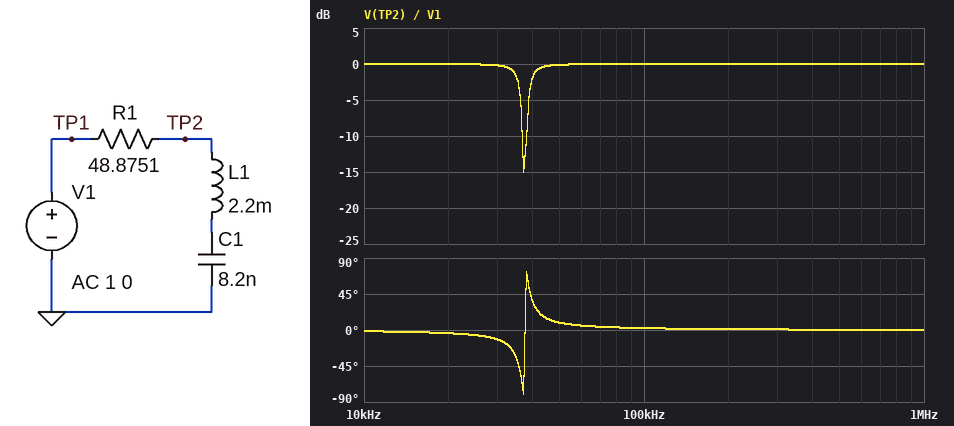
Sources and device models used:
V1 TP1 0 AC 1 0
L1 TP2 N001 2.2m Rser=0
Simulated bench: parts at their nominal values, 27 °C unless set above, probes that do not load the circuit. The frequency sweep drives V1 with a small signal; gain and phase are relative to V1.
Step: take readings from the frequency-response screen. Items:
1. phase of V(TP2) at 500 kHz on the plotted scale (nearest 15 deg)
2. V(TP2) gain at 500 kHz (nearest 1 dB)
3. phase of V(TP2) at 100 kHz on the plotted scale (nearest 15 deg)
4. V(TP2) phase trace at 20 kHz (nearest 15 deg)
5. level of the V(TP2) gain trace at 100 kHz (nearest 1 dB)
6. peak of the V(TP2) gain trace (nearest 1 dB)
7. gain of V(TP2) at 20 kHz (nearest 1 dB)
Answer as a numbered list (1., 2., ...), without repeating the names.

1. 0 deg
2. 0 dB
3. 0 deg
4. 0 deg
5. 0 dB
6. 0 dB
7. 0 dB
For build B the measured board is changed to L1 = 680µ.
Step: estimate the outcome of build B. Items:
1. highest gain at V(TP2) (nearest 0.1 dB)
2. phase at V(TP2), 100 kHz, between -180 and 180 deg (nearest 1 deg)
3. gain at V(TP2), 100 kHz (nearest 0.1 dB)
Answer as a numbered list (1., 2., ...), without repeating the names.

1. 0 dB
2. 12 deg
3. -0.2 dB
